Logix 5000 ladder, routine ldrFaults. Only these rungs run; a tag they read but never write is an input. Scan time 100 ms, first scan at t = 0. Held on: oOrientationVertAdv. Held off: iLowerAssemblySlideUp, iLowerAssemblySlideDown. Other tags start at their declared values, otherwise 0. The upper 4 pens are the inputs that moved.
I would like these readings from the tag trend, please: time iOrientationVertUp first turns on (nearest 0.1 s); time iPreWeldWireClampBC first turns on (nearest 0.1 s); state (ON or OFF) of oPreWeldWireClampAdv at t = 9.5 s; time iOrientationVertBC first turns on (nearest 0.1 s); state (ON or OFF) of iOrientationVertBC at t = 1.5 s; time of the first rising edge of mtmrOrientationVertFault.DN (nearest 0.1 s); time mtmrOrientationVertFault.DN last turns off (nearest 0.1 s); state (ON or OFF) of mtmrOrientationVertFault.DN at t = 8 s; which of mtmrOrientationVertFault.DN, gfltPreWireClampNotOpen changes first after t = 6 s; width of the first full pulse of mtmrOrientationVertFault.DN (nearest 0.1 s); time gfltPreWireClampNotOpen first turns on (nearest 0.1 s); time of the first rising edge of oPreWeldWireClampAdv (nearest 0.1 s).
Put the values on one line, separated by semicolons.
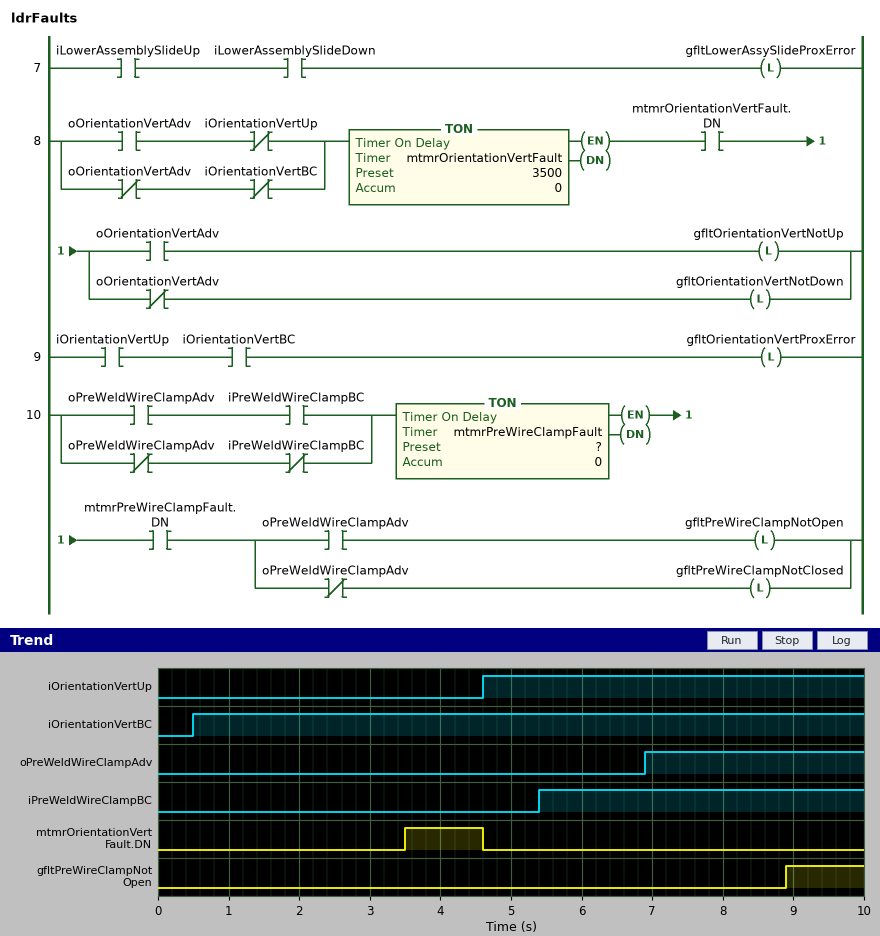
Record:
4.6 s; 5.4 s; ON; 0.5 s; ON; 3.5 s; 4.6 s; OFF; gfltPreWireClampNotOpen; 1.1 s; 8.9 s; 6.9 s
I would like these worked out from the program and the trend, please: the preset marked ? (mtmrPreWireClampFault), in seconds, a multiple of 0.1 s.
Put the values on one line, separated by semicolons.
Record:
2.0 s
